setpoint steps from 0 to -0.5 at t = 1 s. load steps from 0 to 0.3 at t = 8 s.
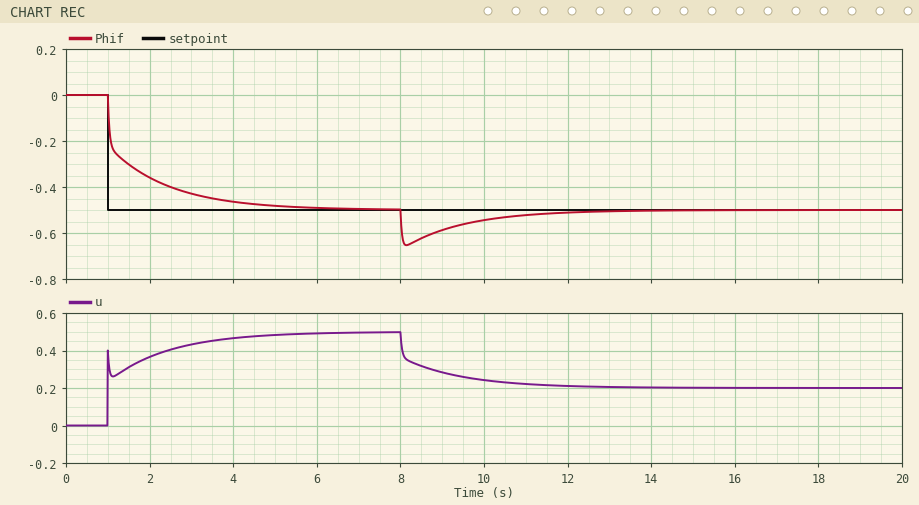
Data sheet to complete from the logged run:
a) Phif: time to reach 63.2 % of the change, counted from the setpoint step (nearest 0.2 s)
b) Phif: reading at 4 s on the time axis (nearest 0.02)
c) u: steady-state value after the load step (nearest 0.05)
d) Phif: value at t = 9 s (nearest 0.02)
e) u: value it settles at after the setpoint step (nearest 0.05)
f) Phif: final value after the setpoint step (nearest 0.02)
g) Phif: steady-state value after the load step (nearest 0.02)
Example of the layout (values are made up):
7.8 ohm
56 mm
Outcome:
0.6 s
-0.46
0.20
-0.58
0.50
-0.50
-0.50
